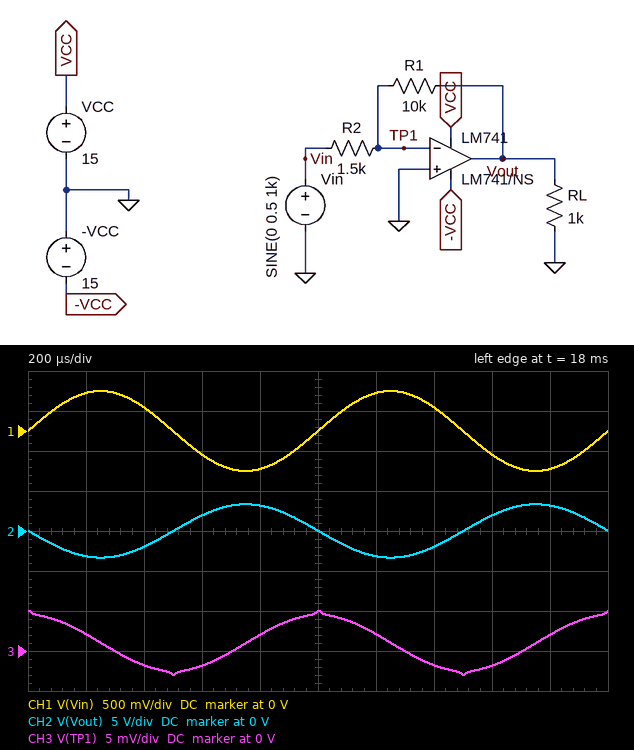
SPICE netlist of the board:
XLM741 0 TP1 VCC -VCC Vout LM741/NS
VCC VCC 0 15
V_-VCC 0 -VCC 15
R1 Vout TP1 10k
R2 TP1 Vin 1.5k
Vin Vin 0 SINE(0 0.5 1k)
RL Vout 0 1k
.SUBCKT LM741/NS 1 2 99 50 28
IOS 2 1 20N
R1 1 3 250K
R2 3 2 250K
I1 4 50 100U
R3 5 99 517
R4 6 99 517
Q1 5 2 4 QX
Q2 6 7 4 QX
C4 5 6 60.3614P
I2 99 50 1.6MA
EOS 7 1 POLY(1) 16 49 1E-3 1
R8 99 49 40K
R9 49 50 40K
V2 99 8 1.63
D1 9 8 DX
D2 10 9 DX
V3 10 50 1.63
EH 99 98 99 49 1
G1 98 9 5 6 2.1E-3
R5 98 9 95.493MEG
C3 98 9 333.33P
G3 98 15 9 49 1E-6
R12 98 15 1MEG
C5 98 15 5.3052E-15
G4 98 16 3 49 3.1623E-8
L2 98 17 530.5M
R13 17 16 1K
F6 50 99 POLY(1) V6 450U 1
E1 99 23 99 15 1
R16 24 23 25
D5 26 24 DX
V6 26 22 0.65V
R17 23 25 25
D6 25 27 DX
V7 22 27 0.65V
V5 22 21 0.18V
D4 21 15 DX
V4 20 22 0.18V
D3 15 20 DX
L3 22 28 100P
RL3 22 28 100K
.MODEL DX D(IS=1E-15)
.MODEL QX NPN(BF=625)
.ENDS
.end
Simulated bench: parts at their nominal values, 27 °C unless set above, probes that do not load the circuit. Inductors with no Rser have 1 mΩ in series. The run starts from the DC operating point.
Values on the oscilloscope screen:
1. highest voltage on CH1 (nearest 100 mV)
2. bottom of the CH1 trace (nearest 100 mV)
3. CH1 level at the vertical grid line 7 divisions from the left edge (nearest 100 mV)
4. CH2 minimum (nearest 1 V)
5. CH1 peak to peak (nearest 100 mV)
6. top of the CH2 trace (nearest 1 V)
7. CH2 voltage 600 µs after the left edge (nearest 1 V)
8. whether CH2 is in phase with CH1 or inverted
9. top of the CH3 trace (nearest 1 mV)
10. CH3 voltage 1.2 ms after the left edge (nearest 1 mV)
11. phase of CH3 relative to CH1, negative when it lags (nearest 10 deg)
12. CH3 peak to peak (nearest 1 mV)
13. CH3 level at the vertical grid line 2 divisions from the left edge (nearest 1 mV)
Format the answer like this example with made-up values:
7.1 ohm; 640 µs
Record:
500 mV; -500 mV; 300 mV; -3 V; 1.0 V; 3 V; 2 V; inverted; 5 mV; 2 mV; 90 deg; 8 mV; -2 mV
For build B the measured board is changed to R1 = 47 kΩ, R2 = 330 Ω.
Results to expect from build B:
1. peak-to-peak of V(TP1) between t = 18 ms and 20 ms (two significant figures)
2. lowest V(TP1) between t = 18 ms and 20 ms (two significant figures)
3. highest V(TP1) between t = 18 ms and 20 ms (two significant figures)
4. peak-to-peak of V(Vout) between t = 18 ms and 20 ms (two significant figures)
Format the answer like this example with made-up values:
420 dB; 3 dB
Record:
800 mV; -400 mV; 400 mV; 27 V
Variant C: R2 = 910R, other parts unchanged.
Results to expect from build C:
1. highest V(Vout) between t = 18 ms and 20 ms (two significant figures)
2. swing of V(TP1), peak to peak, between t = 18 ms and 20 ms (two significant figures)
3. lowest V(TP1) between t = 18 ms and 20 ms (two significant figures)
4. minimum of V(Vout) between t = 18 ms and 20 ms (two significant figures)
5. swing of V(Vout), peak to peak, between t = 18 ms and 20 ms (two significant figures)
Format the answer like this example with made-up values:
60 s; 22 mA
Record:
5.5 V; 13 mV; -5.6 mV; -5.5 V; 11 V
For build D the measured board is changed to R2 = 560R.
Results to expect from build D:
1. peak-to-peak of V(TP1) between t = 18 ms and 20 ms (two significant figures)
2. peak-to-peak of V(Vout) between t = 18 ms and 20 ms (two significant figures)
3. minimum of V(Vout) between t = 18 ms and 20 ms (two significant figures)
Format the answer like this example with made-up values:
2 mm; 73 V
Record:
21 mV; 18 V; -8.9 V
